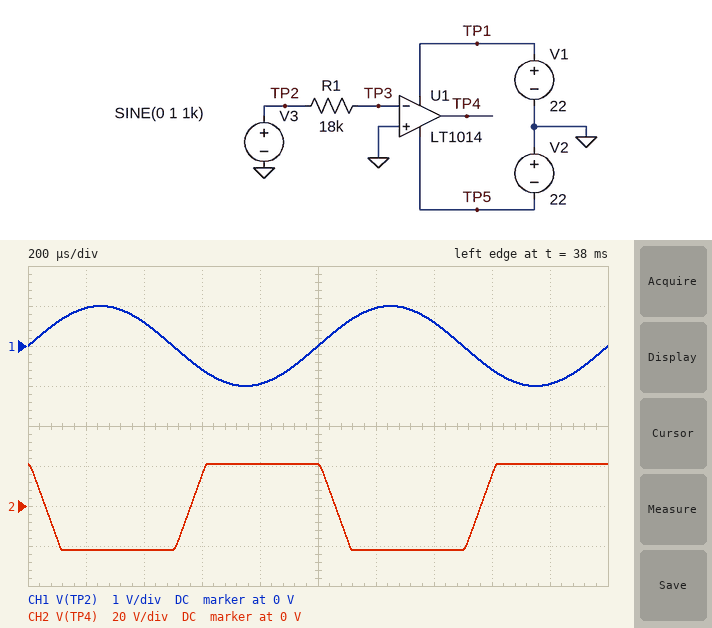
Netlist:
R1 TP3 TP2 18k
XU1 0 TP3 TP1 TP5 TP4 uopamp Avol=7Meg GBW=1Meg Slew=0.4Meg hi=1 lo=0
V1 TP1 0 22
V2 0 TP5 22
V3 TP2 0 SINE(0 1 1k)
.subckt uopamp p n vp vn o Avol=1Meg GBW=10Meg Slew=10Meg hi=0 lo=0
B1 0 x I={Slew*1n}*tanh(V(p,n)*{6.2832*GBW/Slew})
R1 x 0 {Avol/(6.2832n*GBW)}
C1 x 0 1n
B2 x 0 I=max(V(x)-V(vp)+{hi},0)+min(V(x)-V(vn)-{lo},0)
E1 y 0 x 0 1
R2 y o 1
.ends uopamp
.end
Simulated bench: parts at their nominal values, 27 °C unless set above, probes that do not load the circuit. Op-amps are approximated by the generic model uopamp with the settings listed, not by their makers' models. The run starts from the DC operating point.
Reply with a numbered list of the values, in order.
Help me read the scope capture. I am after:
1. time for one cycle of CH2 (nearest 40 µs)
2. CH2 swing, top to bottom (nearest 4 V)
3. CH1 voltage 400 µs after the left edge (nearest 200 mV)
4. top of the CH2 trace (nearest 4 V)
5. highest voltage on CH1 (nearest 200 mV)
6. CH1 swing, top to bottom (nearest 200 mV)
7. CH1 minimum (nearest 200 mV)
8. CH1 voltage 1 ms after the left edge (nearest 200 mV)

1. 1.00 ms
2. 44 V
3. 600 mV
4. 20 V
5. 1.0 V
6. 2.0 V
7. -1.0 V
8. 0 V
